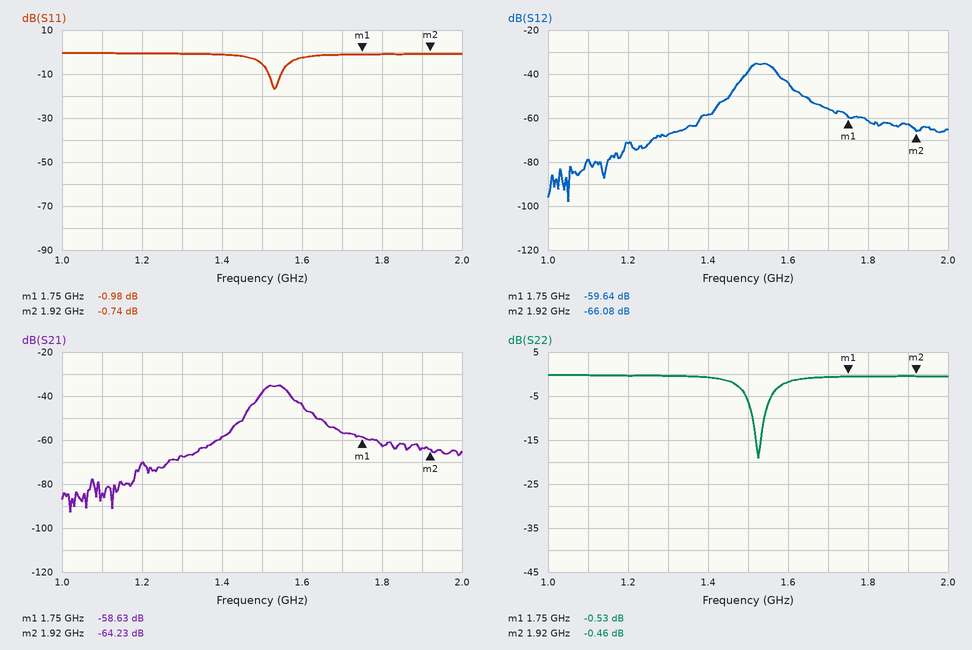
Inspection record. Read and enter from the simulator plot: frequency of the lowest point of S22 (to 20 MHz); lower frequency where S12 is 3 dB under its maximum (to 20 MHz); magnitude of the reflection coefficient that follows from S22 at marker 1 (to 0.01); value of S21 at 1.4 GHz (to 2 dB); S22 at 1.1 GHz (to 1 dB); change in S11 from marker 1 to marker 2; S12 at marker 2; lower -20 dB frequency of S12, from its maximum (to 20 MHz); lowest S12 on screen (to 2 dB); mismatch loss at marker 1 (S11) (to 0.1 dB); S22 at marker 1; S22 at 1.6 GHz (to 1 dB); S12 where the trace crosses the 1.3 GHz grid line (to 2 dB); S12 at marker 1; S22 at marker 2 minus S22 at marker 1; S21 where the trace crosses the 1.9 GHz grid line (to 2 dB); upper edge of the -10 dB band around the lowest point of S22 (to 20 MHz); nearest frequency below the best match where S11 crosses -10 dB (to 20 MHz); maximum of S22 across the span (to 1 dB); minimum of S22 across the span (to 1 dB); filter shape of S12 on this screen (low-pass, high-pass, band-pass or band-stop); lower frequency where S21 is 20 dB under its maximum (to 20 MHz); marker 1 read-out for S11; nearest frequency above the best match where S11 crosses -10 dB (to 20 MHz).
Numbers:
1.52 GHz
1.50 GHz
0.94
-58 dB
0 dB
0.24 dB
-66.08 dB
1.42 GHz
-98 dB
6.9 dB
-0.53 dB
-2 dB
-68 dB
-59.64 dB
0.07 dB
-64 dB
1.54 GHz
1.52 GHz
0 dB
-19 dB
band-pass
1.42 GHz
-0.98 dB
1.54 GHz
